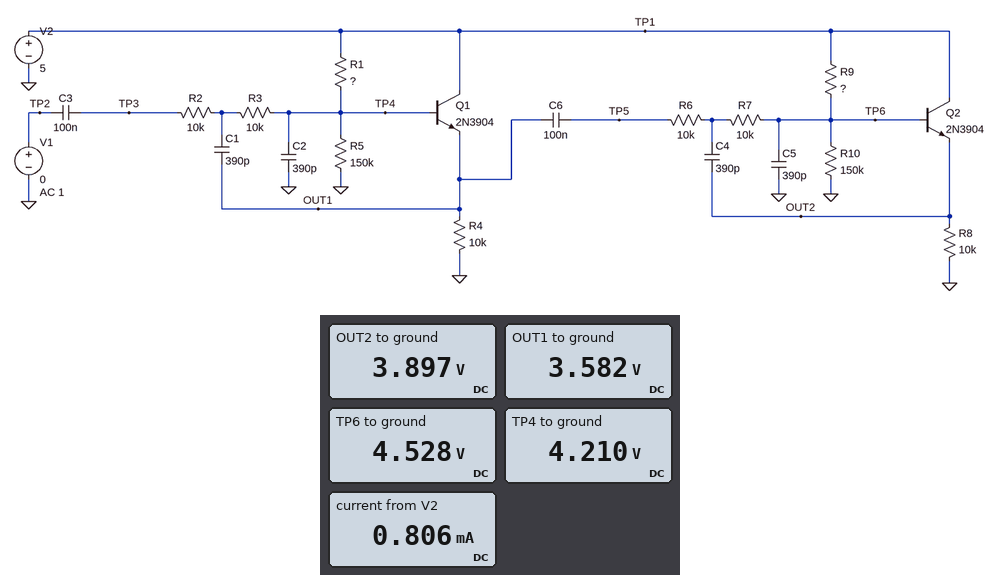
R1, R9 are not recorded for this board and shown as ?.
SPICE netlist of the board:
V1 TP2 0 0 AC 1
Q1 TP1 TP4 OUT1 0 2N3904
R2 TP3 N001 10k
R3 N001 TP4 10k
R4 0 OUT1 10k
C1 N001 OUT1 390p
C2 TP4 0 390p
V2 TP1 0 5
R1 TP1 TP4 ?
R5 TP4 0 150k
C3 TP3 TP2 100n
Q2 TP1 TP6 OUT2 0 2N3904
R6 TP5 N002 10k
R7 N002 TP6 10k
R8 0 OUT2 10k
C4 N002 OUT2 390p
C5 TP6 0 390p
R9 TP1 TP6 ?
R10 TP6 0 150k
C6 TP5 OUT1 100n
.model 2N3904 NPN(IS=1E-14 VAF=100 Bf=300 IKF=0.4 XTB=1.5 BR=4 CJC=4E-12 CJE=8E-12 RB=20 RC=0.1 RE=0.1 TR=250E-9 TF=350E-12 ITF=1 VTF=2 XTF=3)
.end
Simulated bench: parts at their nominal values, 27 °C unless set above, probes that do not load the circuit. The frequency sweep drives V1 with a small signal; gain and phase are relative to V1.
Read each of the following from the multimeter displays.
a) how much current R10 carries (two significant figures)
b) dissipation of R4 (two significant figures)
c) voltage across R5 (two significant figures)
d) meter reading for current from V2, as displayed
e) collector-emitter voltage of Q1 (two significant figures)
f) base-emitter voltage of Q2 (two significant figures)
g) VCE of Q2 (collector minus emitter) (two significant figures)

30 µA
1.3 mW
4.2 V
0.806 mA
1.4 V
630 mV
1.1 V
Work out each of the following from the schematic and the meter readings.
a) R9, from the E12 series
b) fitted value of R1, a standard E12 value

15 kΩ
27 kΩ
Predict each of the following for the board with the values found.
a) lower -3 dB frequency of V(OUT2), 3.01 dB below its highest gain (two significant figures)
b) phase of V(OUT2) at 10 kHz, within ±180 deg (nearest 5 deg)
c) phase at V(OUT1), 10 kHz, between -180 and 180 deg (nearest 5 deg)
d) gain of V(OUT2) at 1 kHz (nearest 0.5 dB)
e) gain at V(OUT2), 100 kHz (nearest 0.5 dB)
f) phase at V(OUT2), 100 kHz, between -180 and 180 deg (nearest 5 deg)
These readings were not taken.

66 Hz
-35 deg
-20 deg
-13.5 dB
-36.0 dB
120 deg
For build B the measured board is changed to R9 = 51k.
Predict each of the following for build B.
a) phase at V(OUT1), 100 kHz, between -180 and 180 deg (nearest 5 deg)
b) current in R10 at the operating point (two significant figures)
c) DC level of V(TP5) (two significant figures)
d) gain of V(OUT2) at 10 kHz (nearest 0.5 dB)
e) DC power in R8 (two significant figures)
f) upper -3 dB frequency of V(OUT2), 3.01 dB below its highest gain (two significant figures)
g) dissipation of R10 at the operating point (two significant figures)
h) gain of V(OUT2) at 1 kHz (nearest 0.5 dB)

-125 deg
25 µA
3.7 V
-10.0 dB
940 µW
27 kHz
91 µW
-9.5 dB
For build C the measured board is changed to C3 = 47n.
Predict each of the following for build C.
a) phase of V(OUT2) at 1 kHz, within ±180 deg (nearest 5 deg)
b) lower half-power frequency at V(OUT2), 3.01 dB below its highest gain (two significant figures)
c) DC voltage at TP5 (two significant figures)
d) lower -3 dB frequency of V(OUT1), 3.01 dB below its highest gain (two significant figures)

5 deg
99 Hz
4.5 V
79 Hz
